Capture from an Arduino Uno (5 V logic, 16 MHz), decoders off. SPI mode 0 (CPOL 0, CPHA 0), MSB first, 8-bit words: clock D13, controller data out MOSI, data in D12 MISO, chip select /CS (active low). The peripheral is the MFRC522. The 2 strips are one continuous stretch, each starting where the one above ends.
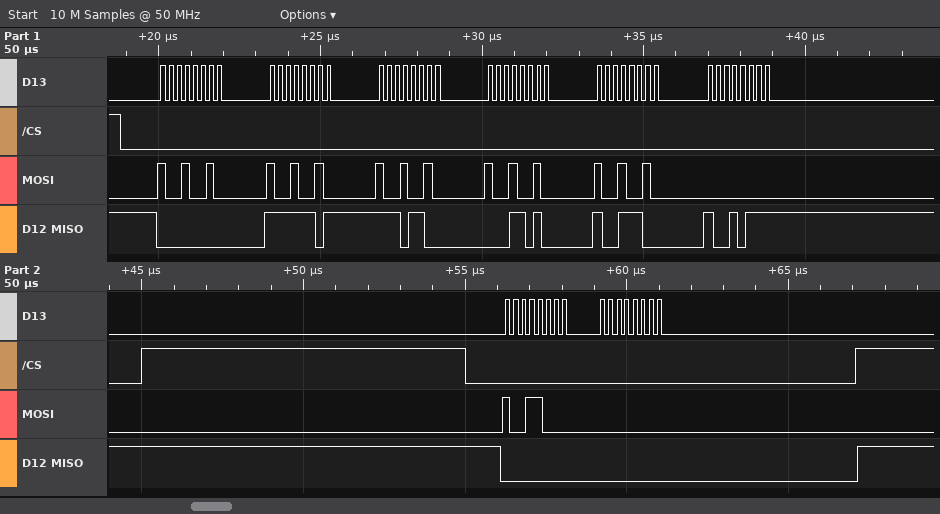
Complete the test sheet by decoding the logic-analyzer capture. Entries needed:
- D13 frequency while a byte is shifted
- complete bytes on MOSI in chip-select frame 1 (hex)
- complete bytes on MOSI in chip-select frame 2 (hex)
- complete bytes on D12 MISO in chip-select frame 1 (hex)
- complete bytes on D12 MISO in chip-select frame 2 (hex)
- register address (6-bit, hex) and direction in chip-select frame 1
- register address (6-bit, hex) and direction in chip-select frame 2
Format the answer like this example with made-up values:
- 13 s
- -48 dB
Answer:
- 4 MHz
- 92 92 92 92 92 00
- 98 00
- 00 FD EC 1A 9C 97
- 00 00
- 0x09 read
- 0x0C read
